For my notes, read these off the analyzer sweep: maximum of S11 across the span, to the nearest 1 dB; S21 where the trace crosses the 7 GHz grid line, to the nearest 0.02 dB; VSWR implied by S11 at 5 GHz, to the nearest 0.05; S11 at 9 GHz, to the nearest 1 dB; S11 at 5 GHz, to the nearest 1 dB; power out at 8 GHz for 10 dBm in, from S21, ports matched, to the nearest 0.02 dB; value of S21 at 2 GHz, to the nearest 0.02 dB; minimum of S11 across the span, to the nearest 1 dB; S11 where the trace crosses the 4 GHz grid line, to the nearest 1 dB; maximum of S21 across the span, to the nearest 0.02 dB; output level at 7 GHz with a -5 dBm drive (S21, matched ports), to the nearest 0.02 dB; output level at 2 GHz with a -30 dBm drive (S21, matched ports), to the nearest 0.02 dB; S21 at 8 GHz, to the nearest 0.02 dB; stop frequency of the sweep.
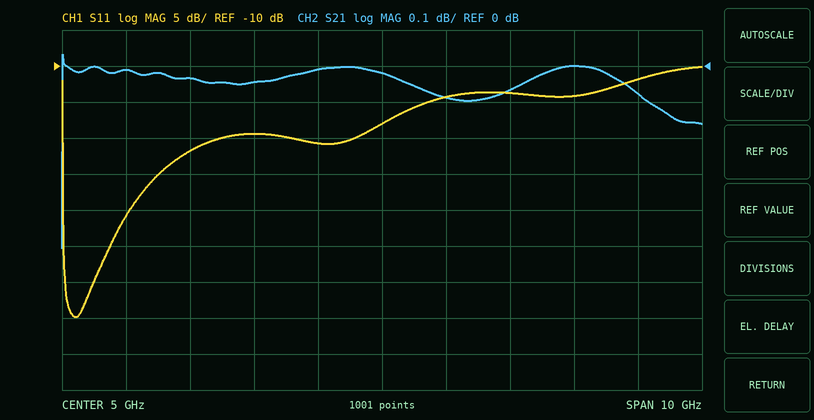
-10 dB
-0.06 dB
1.30
-12 dB
-18 dB
10.00 dBm
-0.04 dB
-45 dB
-21 dB
0.04 dB
-5.06 dBm
-30.04 dBm
0.00 dB
10 GHz
